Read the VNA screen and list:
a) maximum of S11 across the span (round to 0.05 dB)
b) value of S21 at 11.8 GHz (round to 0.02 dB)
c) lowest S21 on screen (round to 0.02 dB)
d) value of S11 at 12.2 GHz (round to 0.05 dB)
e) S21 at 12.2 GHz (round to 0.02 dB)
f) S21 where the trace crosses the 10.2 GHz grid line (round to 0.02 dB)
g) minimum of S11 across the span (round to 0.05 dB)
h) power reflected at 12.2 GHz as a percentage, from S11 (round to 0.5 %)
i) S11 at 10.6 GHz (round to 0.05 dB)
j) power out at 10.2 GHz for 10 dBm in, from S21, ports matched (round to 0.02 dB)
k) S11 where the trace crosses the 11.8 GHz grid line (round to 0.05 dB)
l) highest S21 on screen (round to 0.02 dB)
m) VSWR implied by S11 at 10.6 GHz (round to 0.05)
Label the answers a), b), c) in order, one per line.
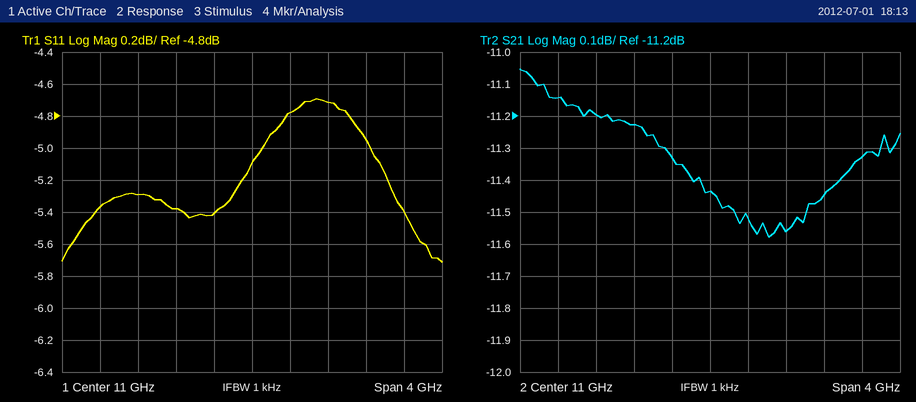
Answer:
a) -4.70 dB
b) -11.56 dB
c) -11.58 dB
d) -4.95 dB
e) -11.44 dB
f) -11.22 dB
g) -5.70 dB
h) 32.0 %
i) -5.40 dB
j) -1.22 dBm
k) -4.70 dB
l) -11.06 dB
m) 3.30
